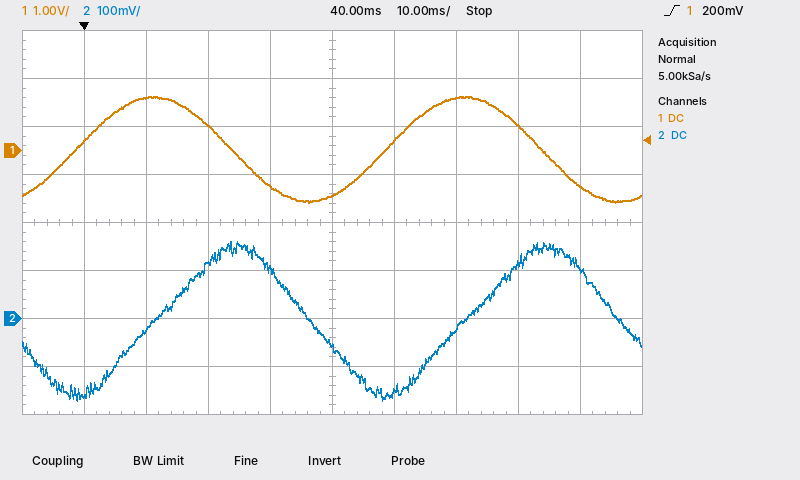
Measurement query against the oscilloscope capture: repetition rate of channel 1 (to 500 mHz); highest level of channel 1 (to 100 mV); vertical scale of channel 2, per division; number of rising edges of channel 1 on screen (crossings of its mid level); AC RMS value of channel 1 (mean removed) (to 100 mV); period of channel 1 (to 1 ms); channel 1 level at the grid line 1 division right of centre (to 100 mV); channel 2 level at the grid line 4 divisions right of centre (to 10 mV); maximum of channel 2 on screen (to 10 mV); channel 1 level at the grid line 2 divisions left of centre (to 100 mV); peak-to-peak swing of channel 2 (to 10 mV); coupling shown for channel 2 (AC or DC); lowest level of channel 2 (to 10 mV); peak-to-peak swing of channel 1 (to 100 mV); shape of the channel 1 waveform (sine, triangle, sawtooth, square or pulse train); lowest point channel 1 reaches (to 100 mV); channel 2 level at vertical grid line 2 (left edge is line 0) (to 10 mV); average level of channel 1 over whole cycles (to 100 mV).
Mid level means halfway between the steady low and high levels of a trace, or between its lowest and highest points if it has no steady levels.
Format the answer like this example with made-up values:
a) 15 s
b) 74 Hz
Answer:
a) 20.0 Hz
b) 1.1 V
c) 100 mV
d) 2
e) 800 mV
f) 50 ms
g) 200 mV
h) 100 mV
i) 160 mV
j) 500 mV
k) 330 mV
l) DC
m) -170 mV
n) 2.2 V
o) sine
p) -1.1 V
q) -20 mV
r) 0.0 V
